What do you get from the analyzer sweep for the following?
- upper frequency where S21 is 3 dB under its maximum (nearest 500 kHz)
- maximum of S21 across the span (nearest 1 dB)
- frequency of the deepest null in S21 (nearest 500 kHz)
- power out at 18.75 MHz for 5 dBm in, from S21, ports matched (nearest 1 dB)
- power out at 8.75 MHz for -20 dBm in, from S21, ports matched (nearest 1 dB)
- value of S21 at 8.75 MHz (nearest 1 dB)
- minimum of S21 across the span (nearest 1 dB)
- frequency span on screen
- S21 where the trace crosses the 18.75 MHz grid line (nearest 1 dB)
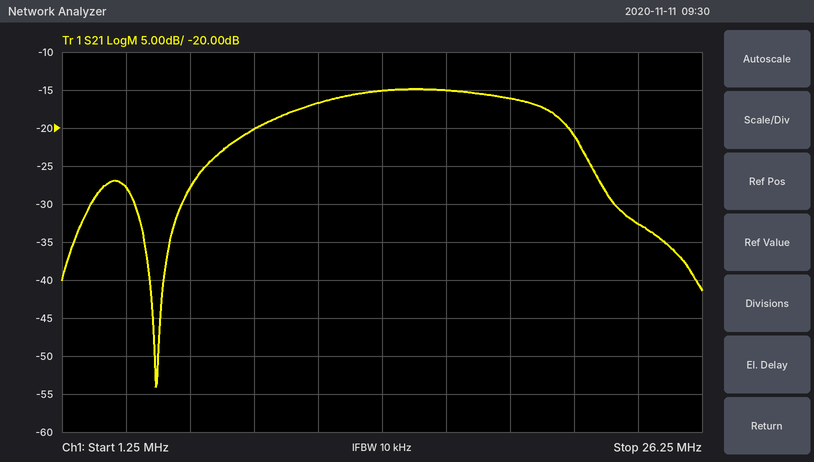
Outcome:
20.5 MHz
-15 dB
5.0 MHz
-11 dBm
-40 dBm
-20 dB
-54 dB
25 MHz
-16 dB
